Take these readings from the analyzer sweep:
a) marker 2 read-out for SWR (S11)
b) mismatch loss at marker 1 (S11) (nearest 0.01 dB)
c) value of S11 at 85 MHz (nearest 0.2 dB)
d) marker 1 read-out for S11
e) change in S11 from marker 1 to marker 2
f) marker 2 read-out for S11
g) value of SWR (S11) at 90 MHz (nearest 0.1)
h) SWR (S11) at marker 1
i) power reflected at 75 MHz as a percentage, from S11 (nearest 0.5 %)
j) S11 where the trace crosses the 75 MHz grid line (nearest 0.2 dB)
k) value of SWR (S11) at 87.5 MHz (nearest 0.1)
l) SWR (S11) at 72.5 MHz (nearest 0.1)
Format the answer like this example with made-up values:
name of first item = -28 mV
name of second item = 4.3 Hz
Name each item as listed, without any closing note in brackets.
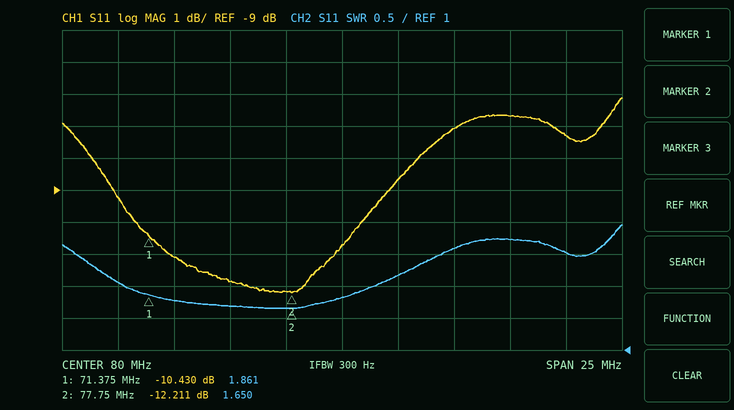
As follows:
marker 2 read-out for SWR = 1.650
mismatch loss at marker 1 (S11) = 0.41 dB
value of S11 at 85 MHz = -7.0 dB
marker 1 read-out for S11 = -10.430 dB
change in S11 from marker 1 to marker 2 = -1.781 dB
marker 2 read-out for S11 = -12.211 dB
value of SWR (S11) at 90 MHz = 2.5
SWR (S11) at marker 1 = 1.861
power reflected at 75 MHz as a percentage, from S11 = 6.5 %
S11 where the trace crosses the 75 MHz grid line = -11.8 dB
value of SWR (S11) at 87.5 MHz = 2.7
SWR (S11) at 72.5 MHz = 1.8
